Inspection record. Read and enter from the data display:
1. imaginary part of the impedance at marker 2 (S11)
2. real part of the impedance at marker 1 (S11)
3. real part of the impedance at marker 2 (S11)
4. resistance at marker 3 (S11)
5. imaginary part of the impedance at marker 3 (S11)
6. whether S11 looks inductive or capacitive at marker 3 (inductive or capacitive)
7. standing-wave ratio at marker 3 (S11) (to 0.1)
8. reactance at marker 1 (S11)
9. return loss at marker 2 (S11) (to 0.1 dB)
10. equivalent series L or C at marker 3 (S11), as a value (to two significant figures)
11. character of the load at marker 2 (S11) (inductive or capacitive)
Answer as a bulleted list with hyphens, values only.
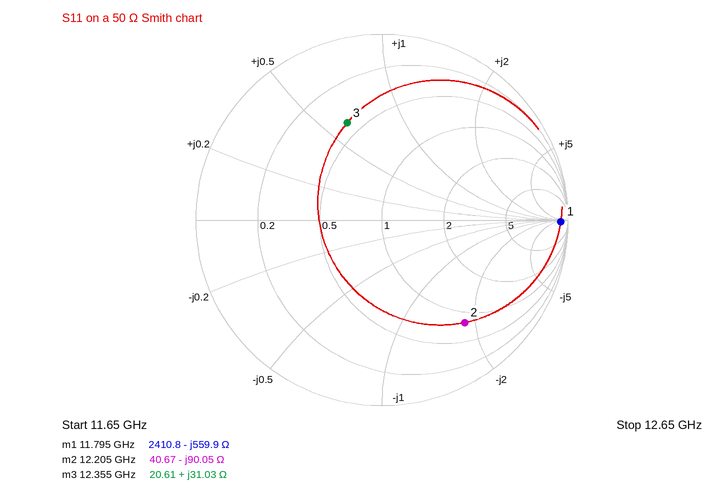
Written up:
- -90.05 Ω
- 2410.8 Ω
- 40.67 Ω
- 20.61 Ω
- +31.03 Ω
- inductive
- 3.5
- -559.9 Ω
- 3.0 dB
- 400 pH
- capacitive
